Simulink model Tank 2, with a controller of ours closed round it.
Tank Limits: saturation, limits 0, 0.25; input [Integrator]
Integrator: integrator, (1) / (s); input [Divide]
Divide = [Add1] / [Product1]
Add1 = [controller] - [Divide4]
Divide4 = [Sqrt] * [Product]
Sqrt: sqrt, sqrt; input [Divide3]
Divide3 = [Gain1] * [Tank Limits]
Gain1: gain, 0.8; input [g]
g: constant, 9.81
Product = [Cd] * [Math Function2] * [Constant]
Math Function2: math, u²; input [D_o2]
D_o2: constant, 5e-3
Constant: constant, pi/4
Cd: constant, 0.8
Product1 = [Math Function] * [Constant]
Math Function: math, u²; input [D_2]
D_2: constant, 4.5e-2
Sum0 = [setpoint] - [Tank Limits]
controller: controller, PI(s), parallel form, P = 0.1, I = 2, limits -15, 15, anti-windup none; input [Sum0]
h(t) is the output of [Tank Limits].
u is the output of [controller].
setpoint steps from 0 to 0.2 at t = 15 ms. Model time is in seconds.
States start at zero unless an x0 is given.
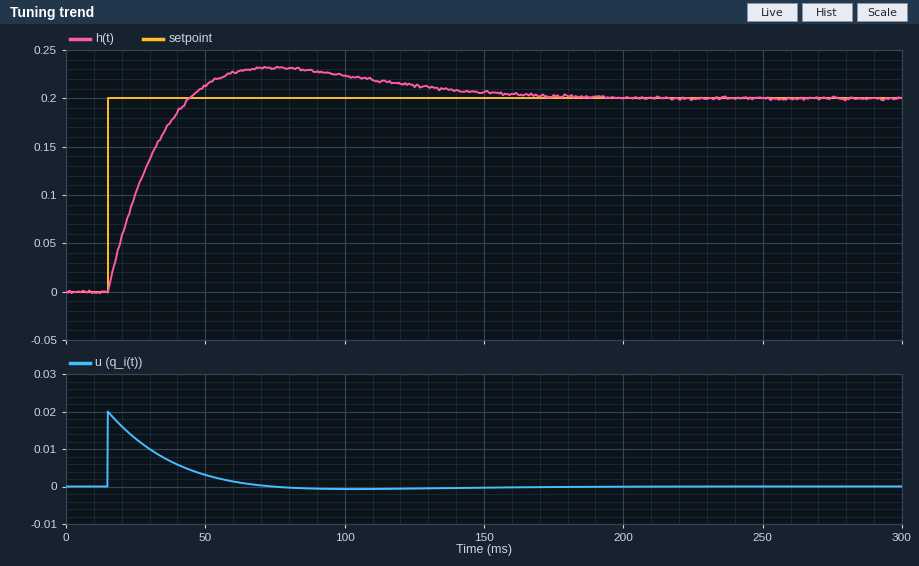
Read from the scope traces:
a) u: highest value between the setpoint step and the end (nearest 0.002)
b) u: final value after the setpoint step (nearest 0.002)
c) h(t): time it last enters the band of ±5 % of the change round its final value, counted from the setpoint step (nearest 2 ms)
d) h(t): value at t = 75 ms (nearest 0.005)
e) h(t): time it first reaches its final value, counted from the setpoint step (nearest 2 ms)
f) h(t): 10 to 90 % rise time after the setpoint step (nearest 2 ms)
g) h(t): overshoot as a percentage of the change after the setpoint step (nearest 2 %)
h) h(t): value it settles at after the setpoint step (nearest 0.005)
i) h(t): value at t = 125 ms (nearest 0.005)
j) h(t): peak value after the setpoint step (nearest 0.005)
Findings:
0.020
0.000
120 ms
0.230
30 ms
22 ms
16 %
0.200
0.215
0.230
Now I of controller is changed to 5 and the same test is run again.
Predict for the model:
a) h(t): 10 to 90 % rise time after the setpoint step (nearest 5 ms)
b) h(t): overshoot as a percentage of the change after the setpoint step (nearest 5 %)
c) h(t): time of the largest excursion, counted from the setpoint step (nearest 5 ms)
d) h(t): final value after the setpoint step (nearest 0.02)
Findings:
15 ms
25 %
35 ms
0.20
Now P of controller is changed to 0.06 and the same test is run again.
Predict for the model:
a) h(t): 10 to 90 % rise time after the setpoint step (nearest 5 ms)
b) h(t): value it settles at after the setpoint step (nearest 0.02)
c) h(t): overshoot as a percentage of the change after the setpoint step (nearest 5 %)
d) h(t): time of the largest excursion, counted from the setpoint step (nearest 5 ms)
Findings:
25 ms
0.20
25 %
55 ms
